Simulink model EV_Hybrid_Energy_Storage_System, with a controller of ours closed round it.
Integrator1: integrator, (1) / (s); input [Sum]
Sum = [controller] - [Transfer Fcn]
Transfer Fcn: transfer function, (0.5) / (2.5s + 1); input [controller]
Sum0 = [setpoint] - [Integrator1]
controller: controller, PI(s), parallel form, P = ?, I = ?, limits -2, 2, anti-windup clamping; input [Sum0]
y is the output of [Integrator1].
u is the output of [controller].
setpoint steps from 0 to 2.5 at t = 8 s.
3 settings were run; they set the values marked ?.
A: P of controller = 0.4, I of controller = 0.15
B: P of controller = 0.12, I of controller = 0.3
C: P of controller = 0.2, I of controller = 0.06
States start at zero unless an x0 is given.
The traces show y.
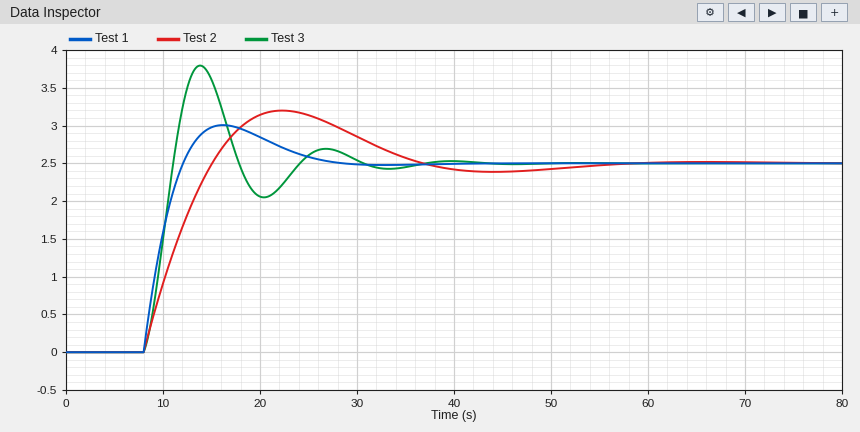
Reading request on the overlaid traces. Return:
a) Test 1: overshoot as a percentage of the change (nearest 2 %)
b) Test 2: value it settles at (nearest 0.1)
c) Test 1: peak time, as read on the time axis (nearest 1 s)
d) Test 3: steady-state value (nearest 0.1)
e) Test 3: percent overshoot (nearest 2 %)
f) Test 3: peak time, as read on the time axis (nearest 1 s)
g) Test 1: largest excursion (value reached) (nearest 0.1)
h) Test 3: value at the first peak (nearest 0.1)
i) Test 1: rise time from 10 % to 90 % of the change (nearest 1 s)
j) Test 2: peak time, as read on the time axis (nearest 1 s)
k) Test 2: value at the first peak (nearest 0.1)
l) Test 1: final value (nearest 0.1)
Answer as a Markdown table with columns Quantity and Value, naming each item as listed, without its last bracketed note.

| Quantity | Value |
|---|---|
| Test 1: overshoot as a percentage of the change | 20 % |
| Test 2: value it settles at | 2.5 |
| Test 1: peak time, as read on the time axis | 16 s |
| Test 3: steady-state value | 2.5 |
| Test 3: percent overshoot | 52 % |
| Test 3: peak time, as read on the time axis | 14 s |
| Test 1: largest excursion (value reached) | 3.0 |
| Test 3: value at the first peak | 3.8 |
| Test 1: rise time from 10 % to 90 % of the change | 3 s |
| Test 2: peak time, as read on the time axis | 22 s |
| Test 2: value at the first peak | 3.2 |
| Test 1: final value | 2.5 |
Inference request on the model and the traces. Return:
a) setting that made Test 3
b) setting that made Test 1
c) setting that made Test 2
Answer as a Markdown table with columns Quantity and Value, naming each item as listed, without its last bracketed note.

| Quantity | Value |
|---|---|
| setting that made Test 3 | B |
| setting that made Test 1 | A |
| setting that made Test 2 | C |
